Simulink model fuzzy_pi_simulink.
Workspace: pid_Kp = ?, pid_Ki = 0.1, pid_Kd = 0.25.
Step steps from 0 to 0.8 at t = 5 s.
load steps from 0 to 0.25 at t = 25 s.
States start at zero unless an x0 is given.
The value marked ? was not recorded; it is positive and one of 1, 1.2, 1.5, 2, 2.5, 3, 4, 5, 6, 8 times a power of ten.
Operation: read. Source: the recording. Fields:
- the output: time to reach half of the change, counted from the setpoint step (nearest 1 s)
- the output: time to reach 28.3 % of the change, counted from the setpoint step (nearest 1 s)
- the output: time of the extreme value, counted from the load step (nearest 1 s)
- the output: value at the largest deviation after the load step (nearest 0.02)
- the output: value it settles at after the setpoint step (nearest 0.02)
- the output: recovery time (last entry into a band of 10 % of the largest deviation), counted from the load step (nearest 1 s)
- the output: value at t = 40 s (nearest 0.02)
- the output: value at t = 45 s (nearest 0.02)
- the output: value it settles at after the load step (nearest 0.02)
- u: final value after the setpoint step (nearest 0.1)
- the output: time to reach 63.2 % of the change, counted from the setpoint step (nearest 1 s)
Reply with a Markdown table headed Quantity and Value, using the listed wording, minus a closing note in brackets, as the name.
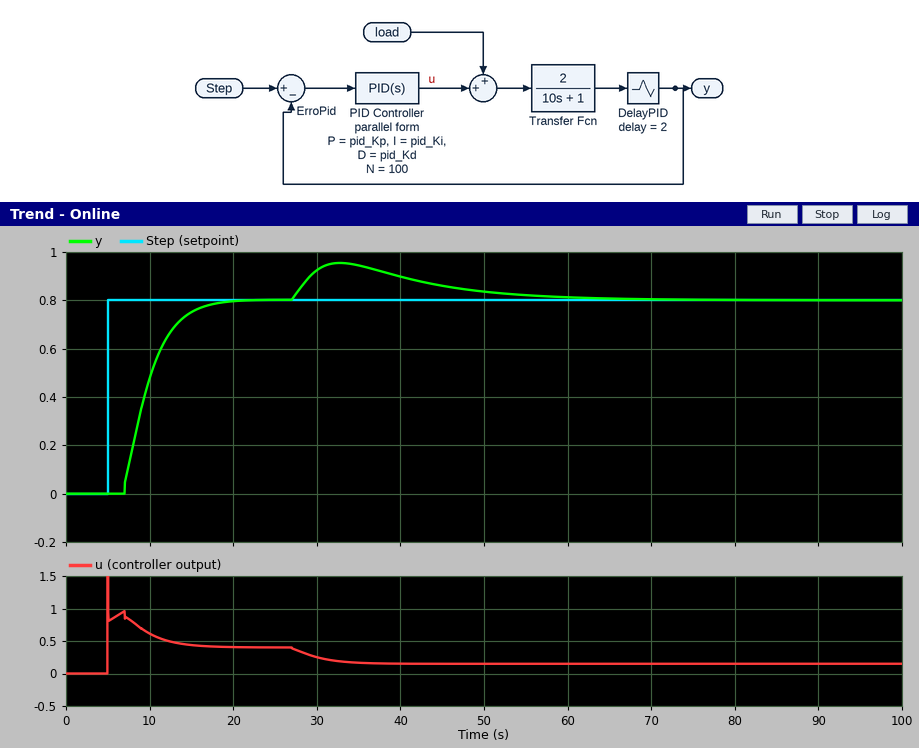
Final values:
| Quantity | Value |
|---|---|
| the output: time to reach half of the change, counted from the setpoint step | 4 s |
| the output: time to reach 28.3 % of the change, counted from the setpoint step | 3 s |
| the output: time of the extreme value, counted from the load step | 8 s |
| the output: value at the largest deviation after the load step | 0.96 |
| the output: value it settles at after the setpoint step | 0.80 |
| the output: recovery time (last entry into a band of 10 % of the largest deviation), counted from the load step | 33 s |
| the output: value at t = 40 s | 0.90 |
| the output: value at t = 45 s | 0.86 |
| the output: value it settles at after the load step | 0.80 |
| u: final value after the setpoint step | 0.4 |
| the output: time to reach 63.2 % of the change, counted from the setpoint step | 5 s |
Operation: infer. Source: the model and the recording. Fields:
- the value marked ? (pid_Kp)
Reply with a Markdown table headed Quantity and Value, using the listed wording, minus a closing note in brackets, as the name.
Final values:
| Quantity | Value |
|---|---|
| the value marked ? | 1 |
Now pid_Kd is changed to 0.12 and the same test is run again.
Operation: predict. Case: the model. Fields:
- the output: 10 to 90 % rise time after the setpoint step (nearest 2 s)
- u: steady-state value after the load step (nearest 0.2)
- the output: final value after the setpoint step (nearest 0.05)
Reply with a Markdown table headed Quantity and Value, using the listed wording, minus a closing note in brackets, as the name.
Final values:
| Quantity | Value |
|---|---|
| the output: 10 to 90 % rise time after the setpoint step | 6 s |
| u: steady-state value after the load step | 0.2 |
| the output: final value after the setpoint step | 0.80 |
